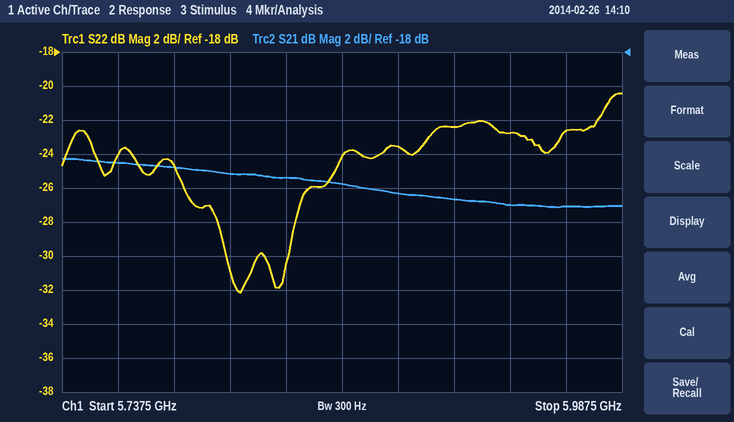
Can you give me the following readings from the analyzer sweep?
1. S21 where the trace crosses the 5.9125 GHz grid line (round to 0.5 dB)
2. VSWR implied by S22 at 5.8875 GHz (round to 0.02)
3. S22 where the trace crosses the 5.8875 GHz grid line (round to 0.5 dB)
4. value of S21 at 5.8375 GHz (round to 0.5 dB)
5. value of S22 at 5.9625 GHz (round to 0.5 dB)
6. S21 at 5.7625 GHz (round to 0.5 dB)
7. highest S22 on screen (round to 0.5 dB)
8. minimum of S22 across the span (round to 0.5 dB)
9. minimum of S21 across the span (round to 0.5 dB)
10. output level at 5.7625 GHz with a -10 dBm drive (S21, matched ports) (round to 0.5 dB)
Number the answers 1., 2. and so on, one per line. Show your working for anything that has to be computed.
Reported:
1. -26.5 dB
2. |Γ| = 10^(-23.5/20) = 0.0668; VSWR = (1 + 0.0668)/(1 − 0.0668) ≈ 1.14
3. -23.5 dB
4. -25.5 dB
5. -22.5 dB
6. -24.5 dB
7. -20.5 dB
8. -32.0 dB
9. -27.0 dB
10. -10 dBm + (-24.5 dB) = -34.5 dBm
